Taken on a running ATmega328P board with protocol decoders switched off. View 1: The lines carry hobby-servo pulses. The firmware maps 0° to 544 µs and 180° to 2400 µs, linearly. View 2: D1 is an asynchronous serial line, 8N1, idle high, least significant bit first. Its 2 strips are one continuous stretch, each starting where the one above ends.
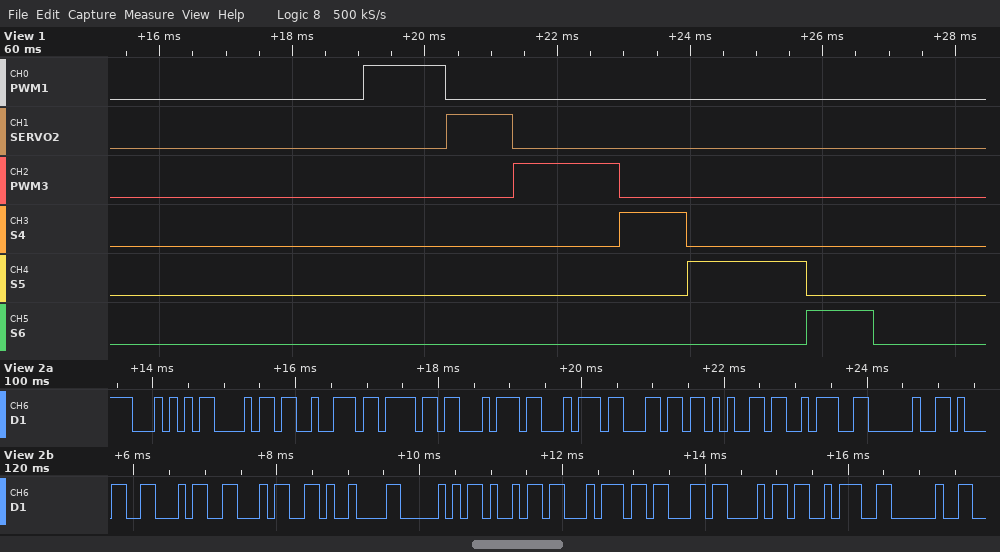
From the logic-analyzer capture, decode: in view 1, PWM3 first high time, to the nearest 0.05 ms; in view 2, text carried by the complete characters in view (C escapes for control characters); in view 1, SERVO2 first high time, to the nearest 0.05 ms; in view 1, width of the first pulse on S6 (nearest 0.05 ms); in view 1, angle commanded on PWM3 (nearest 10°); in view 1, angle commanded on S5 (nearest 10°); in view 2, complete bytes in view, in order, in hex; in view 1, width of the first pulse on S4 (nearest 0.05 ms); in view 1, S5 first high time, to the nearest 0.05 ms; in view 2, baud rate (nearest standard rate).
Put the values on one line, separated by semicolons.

1.60 ms; "Throttle: 144\tPitch: "; 1.00 ms; 1.00 ms; 100°; 120°; 54 68 72 6F 74 74 6C 65 3A 20 31 34 34 09 50 69 74 63 68 3A 20; 1.00 ms; 1.80 ms; 9600 baud
